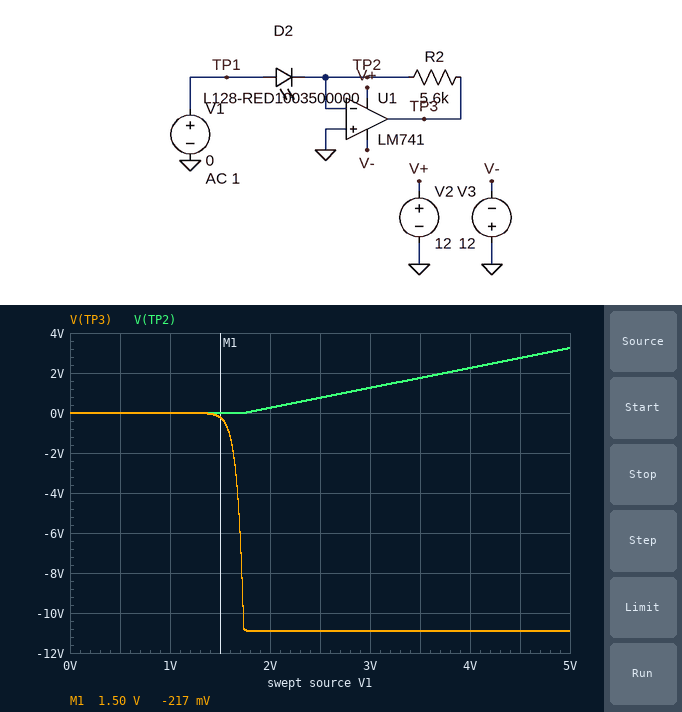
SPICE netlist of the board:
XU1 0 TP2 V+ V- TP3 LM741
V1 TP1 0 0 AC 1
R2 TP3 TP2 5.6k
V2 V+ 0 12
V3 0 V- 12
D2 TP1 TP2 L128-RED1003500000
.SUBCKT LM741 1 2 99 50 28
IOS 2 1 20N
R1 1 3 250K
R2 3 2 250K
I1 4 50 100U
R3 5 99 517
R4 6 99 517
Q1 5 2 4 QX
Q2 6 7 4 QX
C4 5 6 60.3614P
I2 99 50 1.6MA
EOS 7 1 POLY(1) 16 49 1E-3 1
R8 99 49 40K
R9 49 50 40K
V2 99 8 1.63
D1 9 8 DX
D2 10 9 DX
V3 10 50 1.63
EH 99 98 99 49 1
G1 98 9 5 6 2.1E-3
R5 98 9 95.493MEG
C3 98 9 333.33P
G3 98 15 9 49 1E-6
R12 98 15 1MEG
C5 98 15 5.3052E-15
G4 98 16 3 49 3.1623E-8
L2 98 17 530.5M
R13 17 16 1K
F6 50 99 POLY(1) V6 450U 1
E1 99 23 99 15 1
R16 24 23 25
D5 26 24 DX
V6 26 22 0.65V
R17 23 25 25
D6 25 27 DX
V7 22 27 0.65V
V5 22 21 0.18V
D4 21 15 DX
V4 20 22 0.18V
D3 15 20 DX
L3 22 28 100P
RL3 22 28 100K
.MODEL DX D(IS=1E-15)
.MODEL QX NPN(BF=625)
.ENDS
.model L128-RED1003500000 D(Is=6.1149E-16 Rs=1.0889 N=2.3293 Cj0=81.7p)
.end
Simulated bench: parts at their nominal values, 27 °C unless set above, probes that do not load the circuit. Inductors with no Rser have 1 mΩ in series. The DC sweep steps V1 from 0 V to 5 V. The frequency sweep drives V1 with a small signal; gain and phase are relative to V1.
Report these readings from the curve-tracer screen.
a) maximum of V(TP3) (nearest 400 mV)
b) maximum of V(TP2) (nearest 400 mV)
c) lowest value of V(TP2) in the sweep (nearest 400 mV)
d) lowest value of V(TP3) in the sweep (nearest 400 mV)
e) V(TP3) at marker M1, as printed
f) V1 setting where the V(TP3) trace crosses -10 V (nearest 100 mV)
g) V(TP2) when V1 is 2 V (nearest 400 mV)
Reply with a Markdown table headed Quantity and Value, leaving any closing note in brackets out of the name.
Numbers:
| Quantity | Value |
|---|---|
| maximum of V(TP3) | 0 V |
| maximum of V(TP2) | 3.2 V |
| lowest value of V(TP2) in the sweep | 0 V |
| lowest value of V(TP3) in the sweep | -10.8 V |
| V(TP3) at marker M1, as printed | -217 mV |
| V1 setting where the V(TP3) trace crosses -10 V | 1.7 V |
| V(TP2) when V1 is 2 V | 400 mV |
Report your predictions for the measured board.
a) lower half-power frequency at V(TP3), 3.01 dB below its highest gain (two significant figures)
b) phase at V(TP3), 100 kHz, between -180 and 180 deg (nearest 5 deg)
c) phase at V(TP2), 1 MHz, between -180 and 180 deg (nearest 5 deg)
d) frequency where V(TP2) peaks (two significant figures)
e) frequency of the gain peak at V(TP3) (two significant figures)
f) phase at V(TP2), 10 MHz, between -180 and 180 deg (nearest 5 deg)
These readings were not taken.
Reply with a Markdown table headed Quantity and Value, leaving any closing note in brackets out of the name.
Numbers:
| Quantity | Value |
|---|---|
| lower half-power frequency at V(TP3), 3.01 dB below its highest gain | 480 kHz |
| phase at V(TP3), 100 kHz, between -180 and 180 deg | -95 deg |
| phase at V(TP2), 1 MHz, between -180 and 180 deg | 15 deg |
| frequency where V(TP2) peaks | 580 kHz |
| frequency of the gain peak at V(TP3) | 560 kHz |
| phase at V(TP2), 10 MHz, between -180 and 180 deg | 0 deg |
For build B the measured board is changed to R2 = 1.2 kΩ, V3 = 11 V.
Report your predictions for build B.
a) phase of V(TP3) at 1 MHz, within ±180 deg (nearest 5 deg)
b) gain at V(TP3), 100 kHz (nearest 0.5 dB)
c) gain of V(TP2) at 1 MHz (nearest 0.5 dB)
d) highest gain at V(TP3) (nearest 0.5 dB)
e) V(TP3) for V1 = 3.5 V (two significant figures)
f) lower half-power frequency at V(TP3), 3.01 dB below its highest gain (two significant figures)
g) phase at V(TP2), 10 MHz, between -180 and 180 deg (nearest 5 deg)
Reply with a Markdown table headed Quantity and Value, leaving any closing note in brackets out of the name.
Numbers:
| Quantity | Value |
|---|---|
| phase of V(TP3) at 1 MHz, within ±180 deg | 160 deg |
| gain at V(TP3), 100 kHz | -24.0 dB |
| gain of V(TP2) at 1 MHz | 1.5 dB |
| highest gain at V(TP3) | 0.5 dB |
| V(TP3) for V1 = 3.5 V | -9.7 V |
| lower half-power frequency at V(TP3), 3.01 dB below its highest gain | 770 kHz |
| phase at V(TP2), 10 MHz, between -180 and 180 deg | 10 deg |
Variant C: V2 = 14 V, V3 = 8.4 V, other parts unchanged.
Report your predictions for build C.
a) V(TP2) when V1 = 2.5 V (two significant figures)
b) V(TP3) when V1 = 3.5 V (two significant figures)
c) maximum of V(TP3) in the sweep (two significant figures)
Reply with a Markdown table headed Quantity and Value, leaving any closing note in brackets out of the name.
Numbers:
| Quantity | Value |
|---|---|
| V(TP2) when V1 = 2.5 V | 780 mV |
| V(TP3) when V1 = 3.5 V | -7.3 V |
| maximum of V(TP3) in the sweep | 1.5 mV |
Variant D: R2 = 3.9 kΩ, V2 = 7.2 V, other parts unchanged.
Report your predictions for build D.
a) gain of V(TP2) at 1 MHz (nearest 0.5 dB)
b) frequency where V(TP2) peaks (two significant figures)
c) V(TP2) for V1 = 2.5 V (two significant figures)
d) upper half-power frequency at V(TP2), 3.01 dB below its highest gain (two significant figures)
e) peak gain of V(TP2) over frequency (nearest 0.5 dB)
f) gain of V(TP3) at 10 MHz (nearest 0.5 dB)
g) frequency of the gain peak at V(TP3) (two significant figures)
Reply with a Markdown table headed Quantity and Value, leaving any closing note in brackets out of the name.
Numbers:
| Quantity | Value |
|---|---|
| gain of V(TP2) at 1 MHz | 3.5 dB |
| frequency where V(TP2) peaks | 690 kHz |
| V(TP2) for V1 = 2.5 V | 740 mV |
| upper half-power frequency at V(TP2), 3.01 dB below its highest gain | 890 kHz |
| peak gain of V(TP2) over frequency | 8.0 dB |
| gain of V(TP3) at 10 MHz | -23.5 dB |
| frequency of the gain peak at V(TP3) | 660 kHz |
